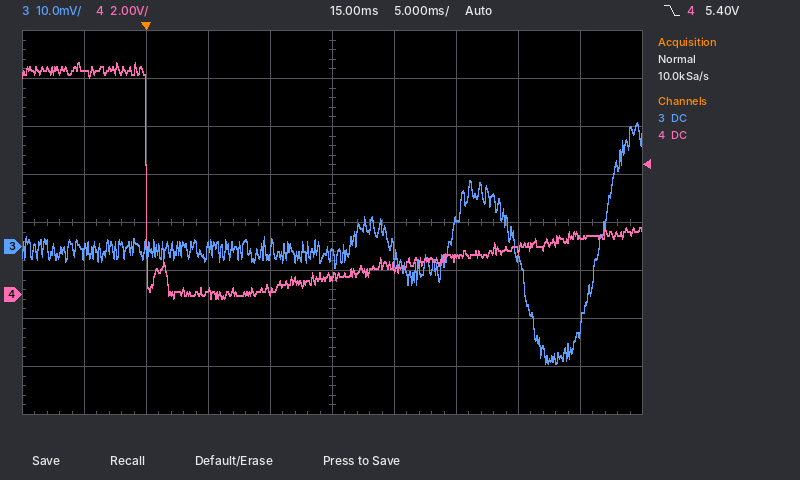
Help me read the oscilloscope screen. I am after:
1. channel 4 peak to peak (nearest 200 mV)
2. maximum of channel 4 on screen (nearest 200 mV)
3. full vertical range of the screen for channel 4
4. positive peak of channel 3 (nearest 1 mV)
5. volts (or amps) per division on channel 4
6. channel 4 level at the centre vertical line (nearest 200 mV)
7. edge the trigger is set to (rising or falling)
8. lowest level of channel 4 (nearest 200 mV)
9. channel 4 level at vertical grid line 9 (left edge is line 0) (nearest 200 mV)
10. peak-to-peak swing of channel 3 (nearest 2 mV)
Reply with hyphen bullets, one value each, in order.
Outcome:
- 9.8 V
- 9.6 V
- 16 V
- 26 mV
- 2 V
- 800 mV
- falling
- -200 mV
- 2.4 V
- 50 mV
